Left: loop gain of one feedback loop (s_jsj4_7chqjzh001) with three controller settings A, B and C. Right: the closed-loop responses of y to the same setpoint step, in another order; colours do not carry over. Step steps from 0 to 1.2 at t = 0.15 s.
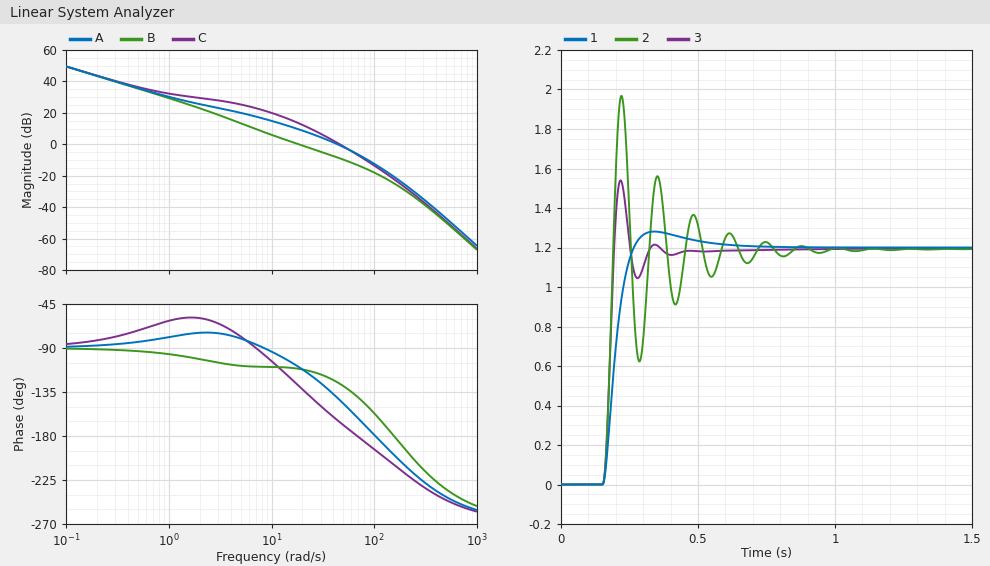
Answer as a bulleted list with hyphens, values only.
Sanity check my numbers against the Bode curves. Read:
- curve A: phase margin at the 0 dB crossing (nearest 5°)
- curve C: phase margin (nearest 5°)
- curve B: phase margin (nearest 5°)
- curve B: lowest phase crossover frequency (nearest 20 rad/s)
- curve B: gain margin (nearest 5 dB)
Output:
- 40°
- 15°
- 70°
- 160 rad/s
- 25 dB
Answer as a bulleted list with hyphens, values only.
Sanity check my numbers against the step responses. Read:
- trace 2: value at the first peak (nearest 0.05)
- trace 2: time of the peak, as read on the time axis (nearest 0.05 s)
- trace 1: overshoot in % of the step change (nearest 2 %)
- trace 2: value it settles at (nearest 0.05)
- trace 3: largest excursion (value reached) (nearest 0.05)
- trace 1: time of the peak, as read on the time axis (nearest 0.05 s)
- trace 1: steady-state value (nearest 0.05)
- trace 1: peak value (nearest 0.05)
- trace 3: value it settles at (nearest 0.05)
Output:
- 1.95
- 0.20 s
- 6 %
- 1.20
- 1.55
- 0.35 s
- 1.20
- 1.30
- 1.20
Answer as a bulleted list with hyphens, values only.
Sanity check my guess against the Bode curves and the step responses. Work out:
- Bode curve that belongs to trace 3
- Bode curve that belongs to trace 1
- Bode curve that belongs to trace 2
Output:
- A
- B
- C
